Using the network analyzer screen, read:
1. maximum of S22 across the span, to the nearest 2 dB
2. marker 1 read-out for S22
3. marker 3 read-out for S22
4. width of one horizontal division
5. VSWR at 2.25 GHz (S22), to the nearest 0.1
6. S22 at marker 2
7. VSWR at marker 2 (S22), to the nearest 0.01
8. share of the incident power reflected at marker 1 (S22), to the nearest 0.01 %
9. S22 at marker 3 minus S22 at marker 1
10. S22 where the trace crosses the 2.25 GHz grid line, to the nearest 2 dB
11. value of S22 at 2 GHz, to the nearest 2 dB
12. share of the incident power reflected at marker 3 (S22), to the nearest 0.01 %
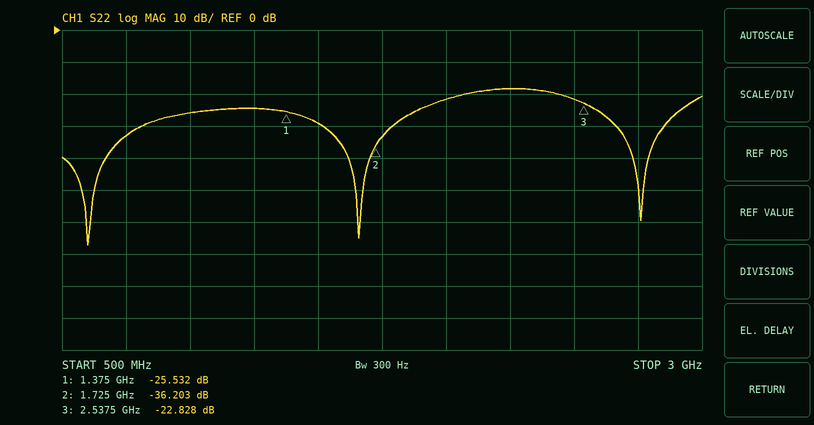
-18 dB
-25.532 dB
-22.828 dB
250 MHz
1.3
-36.203 dB
1.03
0.28 %
2.704 dB
-18 dB
-22 dB
0.52 %
